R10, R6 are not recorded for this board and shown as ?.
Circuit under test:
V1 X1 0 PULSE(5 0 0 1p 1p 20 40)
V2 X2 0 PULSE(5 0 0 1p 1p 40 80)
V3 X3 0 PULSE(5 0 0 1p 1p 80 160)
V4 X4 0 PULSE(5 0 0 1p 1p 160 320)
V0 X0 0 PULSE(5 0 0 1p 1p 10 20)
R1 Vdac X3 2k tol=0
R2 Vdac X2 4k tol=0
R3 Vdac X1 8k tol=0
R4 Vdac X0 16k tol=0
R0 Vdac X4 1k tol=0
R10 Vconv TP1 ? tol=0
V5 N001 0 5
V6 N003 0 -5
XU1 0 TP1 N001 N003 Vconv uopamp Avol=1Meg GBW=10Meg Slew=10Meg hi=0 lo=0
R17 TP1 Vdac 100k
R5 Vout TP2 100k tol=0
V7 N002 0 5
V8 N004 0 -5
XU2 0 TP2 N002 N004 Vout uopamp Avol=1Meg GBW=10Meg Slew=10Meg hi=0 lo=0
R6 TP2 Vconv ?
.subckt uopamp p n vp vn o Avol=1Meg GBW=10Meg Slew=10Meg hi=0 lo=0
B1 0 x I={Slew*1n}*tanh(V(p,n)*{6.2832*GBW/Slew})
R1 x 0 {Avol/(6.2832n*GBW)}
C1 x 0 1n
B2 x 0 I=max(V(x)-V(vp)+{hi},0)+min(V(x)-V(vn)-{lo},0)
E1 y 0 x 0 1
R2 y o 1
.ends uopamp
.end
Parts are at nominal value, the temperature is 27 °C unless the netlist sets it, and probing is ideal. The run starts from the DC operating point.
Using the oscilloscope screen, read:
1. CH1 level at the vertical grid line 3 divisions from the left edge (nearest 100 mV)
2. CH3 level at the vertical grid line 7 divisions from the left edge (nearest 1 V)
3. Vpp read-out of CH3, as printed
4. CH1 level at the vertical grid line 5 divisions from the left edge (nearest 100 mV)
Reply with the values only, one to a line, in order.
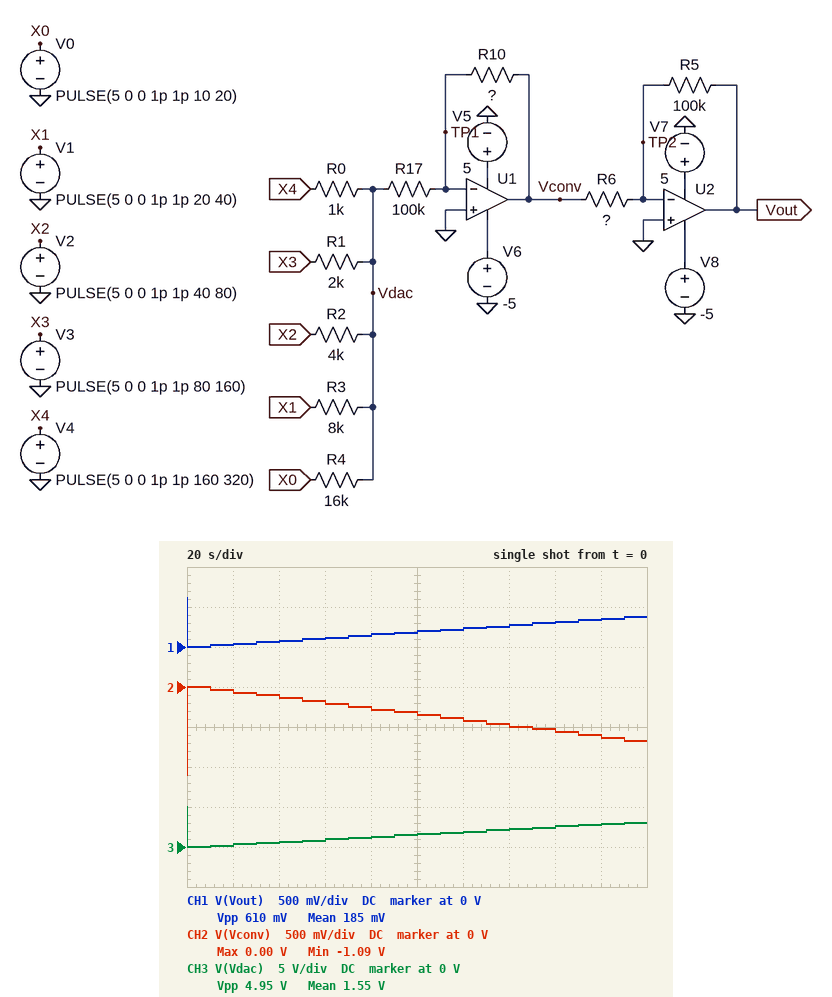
100 mV
2 V
4.95 V
200 mV
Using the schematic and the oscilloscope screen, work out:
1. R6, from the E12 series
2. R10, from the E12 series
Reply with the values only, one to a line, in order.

180 kΩ
22 kΩ
